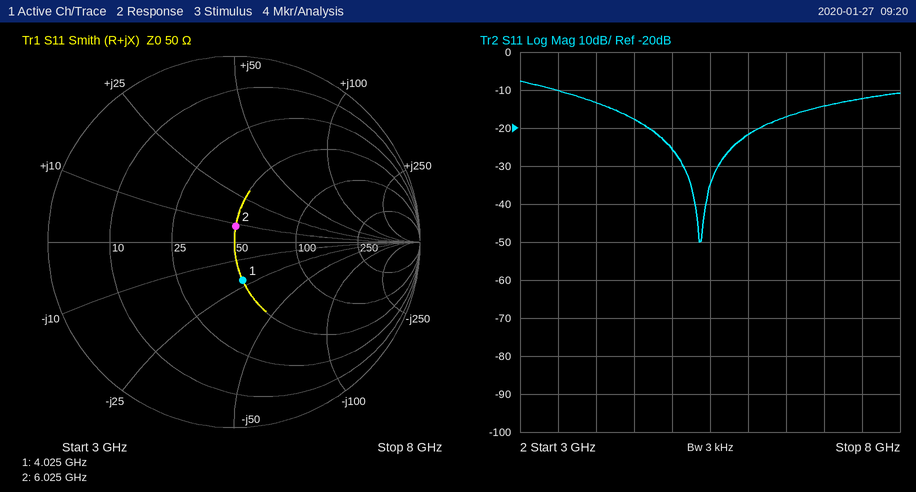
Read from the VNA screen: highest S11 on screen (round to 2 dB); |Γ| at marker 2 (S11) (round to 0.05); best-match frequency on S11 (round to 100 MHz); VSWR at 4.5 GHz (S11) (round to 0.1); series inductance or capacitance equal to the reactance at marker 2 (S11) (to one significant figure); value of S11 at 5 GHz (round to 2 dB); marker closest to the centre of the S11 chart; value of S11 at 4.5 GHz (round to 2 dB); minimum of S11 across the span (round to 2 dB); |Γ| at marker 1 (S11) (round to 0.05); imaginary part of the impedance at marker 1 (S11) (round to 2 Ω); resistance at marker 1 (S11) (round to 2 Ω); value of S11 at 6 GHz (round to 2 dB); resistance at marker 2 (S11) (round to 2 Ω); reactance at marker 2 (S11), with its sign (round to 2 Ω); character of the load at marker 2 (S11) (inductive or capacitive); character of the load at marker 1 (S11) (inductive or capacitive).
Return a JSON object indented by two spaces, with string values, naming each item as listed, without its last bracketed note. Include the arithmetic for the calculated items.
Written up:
{
  "highest S11 on screen": "-8 dB",
  "|Γ| at marker 2 (S11)": "0.10",
  "best-match frequency on S11": "5.4 GHz",
  "VSWR at 4.5 GHz (S11)": "|Γ| = 10^(-18/20) = 0.1259; VSWR = (1 + 0.1259)/(1 − 0.1259) ≈ 1.3",
  "series inductance or capacitance equal to the reactance at marker 2 (S11)": "L = 8 Ω/(2π × 6.025 GHz) ≈ 211 pH, so 200 pH to one significant figure",
  "value of S11 at 5 GHz": "-26 dB",
  "marker closest to the centre of the S11 chart": "marker 2",
  "value of S11 at 4.5 GHz": "-18 dB",
  "minimum of S11 across the span": "-50 dB",
  "|Γ| at marker 1 (S11)": "0.20",
  "imaginary part of the impedance at marker 1 (S11)": "-22 Ω",
  "resistance at marker 1 (S11)": "50 Ω",
  "value of S11 at 6 GHz": "-22 dB",
  "resistance at marker 2 (S11)": "50 Ω",
  "reactance at marker 2 (S11), with its sign": "+8 Ω",
  "character of the load at marker 2 (S11)": "inductive",
  "character of the load at marker 1 (S11)": "capacitive"
}
